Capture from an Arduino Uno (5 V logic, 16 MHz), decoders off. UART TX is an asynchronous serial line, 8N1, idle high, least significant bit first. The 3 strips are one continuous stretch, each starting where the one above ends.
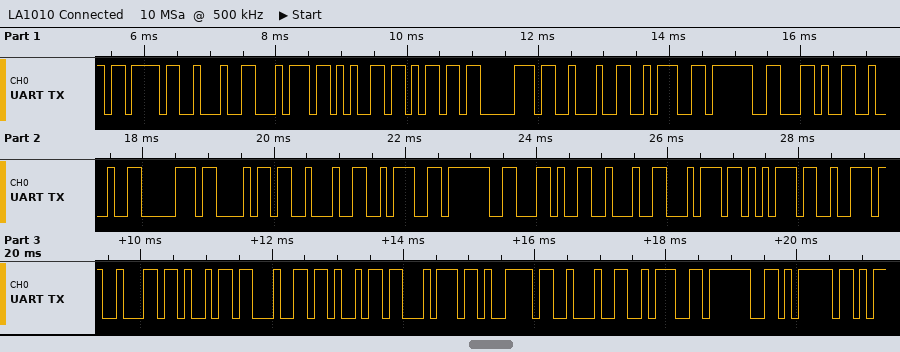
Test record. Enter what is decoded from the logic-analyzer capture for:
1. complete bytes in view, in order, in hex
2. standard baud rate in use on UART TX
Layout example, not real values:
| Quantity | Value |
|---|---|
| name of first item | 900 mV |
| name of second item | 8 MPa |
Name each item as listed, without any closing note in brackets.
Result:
| Quantity | Value |
|---|---|
| complete bytes in view, in order, in hex | 0x7B 0x22 0x74 0x65 0x6D 0x70 0x22 0x3A 0x3F 0x2C 0x22 0x70 0x68 0x22 0x3A 0x3F 0x2C 0x22 0x74 0x75 0x72 0x62 0x69 0x64 0x69 0x74 0x79 0x22 0x3A 0x3F 0x7D |
| standard baud rate in use on UART TX | 9600 baud |
